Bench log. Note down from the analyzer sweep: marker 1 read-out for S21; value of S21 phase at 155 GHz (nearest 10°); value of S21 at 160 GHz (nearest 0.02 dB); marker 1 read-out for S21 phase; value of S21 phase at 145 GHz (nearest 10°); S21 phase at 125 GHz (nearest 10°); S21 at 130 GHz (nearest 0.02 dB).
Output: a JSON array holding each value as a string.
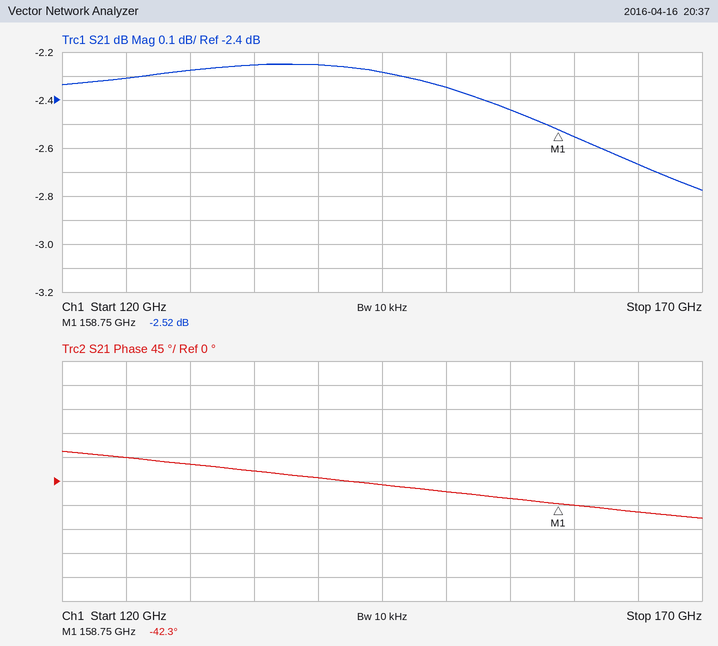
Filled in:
["-2.52 dB", "-30°", "-2.56 dB", "-42.3°", "-10°", "40°", "-2.28 dB"]
